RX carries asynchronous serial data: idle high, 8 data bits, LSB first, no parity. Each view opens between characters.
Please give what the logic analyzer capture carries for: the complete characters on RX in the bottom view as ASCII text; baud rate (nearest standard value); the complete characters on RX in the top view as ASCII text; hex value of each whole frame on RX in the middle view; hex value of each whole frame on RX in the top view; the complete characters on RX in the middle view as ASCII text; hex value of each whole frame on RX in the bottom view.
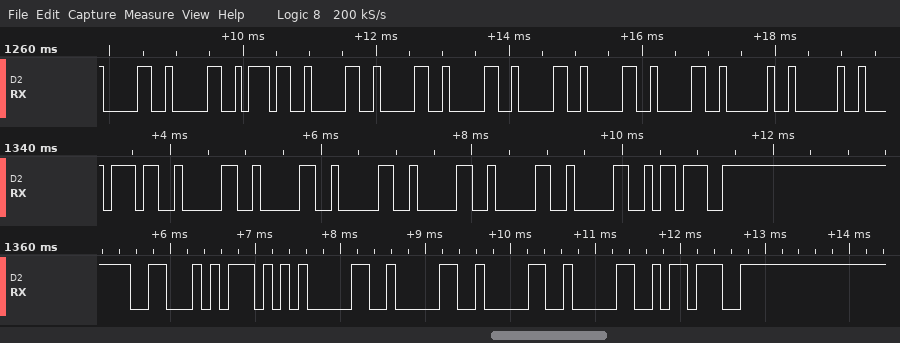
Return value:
"FW0000;"
9600 baud
"007000000  "
37, 30, 30, 30, 30, 30, 30, 3B
30, 30, 37, 30, 30, 30, 30, 30, 30, 20, 20
"7000000;"
46, 57, 30, 30, 30, 30, 3B
